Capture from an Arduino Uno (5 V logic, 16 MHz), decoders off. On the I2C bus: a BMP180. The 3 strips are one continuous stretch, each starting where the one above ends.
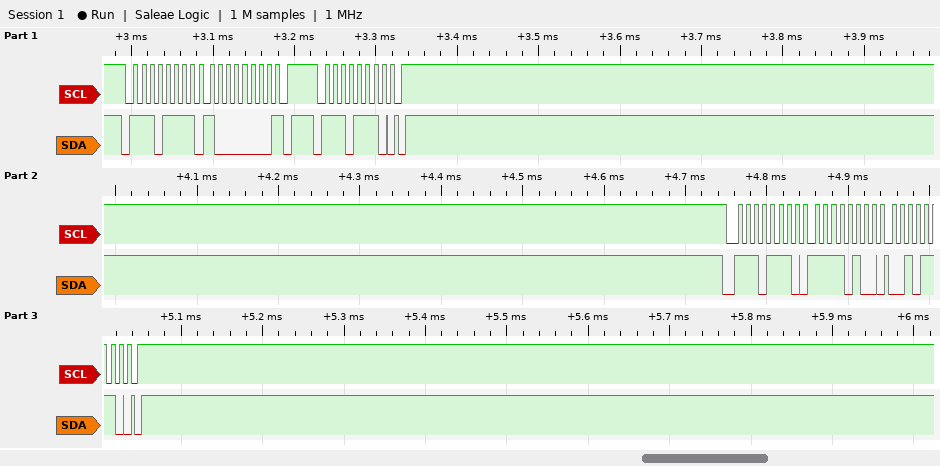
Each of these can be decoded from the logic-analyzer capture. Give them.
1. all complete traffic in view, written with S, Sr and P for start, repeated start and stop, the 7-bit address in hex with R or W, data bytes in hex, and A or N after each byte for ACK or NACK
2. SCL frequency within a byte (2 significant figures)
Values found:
S 77R A 80 N P S 77W A P S 77W A F4 A 2E A P
100 kHz
